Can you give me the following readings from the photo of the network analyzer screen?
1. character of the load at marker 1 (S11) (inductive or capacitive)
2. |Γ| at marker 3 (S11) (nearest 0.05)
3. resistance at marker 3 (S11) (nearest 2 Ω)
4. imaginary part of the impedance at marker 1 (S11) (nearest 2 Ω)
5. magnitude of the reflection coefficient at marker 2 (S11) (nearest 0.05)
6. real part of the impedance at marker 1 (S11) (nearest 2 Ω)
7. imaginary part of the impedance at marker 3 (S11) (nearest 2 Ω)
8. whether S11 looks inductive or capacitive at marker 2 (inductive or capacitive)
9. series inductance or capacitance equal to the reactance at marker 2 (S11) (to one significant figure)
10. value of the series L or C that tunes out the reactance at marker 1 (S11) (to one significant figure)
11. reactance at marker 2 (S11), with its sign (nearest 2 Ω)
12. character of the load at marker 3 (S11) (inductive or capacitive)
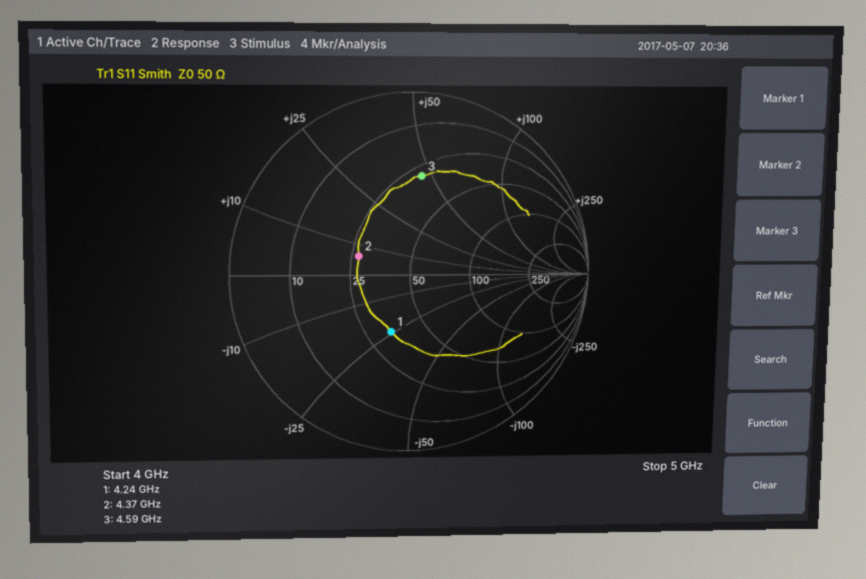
capacitive
0.55
30 Ω
-24 Ω
0.30
34 Ω
+46 Ω
inductive
200 pH
900 pH
+6 Ω
inductive
